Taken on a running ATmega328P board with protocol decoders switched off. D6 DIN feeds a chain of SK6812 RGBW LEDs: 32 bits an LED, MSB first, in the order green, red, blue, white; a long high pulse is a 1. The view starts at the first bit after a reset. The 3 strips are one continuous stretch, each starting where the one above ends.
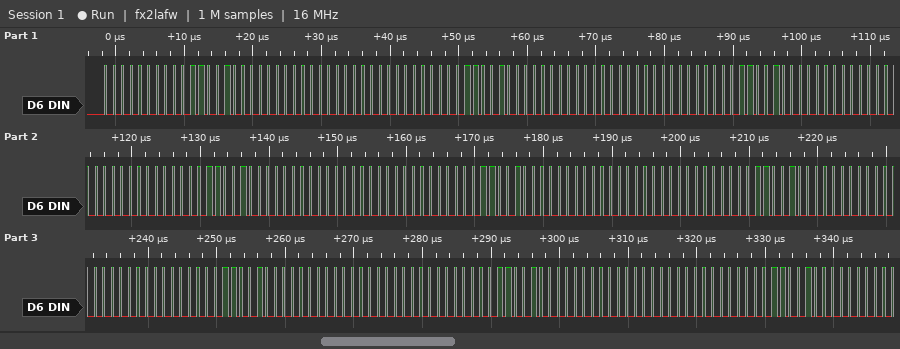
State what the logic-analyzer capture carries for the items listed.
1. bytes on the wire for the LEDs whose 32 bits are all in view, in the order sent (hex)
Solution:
00 32 00 00 00 32 00 00 00 32 00 00 00 32 00 00 00 32 00 00 00 32 00 00 00 32 00 00 00 32 00 00
